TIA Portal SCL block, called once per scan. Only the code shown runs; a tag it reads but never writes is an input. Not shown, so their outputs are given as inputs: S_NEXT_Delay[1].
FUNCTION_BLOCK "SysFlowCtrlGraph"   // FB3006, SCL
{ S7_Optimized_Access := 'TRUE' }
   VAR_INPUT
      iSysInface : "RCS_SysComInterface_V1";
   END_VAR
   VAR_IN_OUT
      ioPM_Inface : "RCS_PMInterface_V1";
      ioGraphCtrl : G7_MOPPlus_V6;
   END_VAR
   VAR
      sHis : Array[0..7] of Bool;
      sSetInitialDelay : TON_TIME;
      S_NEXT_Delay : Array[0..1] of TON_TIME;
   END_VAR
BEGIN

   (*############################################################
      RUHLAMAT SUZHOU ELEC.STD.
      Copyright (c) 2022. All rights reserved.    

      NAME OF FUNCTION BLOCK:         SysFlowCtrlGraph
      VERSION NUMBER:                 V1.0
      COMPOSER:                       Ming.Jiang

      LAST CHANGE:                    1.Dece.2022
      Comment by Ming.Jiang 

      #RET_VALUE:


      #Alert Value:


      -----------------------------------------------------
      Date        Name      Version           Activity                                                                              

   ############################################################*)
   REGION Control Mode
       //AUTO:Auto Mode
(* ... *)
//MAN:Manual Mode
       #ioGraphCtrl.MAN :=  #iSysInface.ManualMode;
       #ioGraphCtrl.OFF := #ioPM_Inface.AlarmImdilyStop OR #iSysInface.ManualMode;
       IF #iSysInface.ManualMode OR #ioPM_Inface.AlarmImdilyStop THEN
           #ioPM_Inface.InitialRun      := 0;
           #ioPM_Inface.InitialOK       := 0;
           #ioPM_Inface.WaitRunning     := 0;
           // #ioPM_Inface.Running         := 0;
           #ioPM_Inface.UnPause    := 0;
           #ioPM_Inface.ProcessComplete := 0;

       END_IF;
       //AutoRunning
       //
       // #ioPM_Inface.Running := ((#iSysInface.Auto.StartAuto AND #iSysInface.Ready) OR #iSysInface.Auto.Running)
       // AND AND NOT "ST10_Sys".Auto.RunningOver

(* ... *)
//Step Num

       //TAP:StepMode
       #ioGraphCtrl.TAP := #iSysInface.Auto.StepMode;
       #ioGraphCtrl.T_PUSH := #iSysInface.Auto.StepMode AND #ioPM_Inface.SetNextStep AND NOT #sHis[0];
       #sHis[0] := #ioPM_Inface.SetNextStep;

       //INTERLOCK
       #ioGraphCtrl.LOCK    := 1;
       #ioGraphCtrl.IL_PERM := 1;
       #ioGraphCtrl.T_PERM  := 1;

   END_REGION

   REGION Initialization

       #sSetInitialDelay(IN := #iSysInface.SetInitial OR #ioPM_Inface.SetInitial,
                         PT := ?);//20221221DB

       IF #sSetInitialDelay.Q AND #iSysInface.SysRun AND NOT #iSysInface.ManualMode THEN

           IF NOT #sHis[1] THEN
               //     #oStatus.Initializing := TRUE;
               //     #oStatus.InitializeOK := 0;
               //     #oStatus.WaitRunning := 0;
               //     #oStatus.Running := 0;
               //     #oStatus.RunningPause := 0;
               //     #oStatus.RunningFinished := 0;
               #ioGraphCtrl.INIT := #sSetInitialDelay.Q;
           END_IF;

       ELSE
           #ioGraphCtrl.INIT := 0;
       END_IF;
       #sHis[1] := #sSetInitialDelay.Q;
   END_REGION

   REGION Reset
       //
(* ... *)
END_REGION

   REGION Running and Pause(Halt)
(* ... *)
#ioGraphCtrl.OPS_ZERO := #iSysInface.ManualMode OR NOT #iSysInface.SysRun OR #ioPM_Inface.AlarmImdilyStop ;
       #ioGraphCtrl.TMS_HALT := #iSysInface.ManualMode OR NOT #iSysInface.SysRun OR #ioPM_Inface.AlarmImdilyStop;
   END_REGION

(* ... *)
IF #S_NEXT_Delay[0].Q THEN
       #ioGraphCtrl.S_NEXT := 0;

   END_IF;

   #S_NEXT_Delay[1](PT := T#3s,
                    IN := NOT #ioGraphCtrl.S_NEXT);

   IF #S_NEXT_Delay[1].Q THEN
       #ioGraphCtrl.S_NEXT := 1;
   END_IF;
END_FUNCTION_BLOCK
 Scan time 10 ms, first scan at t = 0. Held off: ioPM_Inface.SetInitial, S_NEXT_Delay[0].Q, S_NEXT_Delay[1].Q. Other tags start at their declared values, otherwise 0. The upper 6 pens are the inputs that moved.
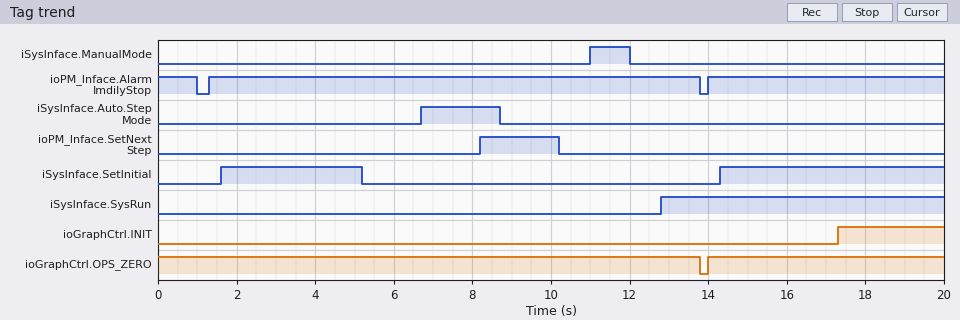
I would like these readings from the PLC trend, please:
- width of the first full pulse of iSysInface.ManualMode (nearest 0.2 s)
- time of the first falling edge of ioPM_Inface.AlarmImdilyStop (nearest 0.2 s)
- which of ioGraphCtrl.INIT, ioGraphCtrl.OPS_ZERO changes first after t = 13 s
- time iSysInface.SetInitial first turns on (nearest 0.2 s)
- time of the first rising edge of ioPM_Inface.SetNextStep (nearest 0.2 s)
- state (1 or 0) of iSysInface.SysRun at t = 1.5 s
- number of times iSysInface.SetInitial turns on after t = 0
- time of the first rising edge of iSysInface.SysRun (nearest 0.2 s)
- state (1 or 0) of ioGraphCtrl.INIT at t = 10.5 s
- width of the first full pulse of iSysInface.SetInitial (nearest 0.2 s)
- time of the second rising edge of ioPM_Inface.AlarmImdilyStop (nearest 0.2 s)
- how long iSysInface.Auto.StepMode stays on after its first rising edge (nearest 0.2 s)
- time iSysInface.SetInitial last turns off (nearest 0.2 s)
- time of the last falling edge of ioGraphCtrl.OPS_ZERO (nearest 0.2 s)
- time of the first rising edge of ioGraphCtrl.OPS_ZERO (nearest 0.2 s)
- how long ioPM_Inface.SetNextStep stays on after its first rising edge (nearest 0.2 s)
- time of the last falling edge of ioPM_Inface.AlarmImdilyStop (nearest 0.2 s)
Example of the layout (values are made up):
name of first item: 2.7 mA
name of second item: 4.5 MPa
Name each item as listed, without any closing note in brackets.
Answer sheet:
width of the first full pulse of iSysInface.ManualMode: 1.0 s
time of the first falling edge of ioPM_Inface.AlarmImdilyStop: 1.0 s
which of ioGraphCtrl.INIT, ioGraphCtrl.OPS_ZERO changes first after t = 13 s: ioGraphCtrl.OPS_ZERO
time iSysInface.SetInitial first turns on: 1.6 s
time of the first rising edge of ioPM_Inface.SetNextStep: 8.2 s
state (1 or 0) of iSysInface.SysRun at t = 1.5 s: 0
number of times iSysInface.SetInitial turns on after t = 0: 2
time of the first rising edge of iSysInface.SysRun: 12.8 s
state (1 or 0) of ioGraphCtrl.INIT at t = 10.5 s: 0
width of the first full pulse of iSysInface.SetInitial: 3.6 s
time of the second rising edge of ioPM_Inface.AlarmImdilyStop: 14.0 s
how long iSysInface.Auto.StepMode stays on after its first rising edge: 2.0 s
time iSysInface.SetInitial last turns off: 5.2 s
time of the last falling edge of ioGraphCtrl.OPS_ZERO: 13.8 s
time of the first rising edge of ioGraphCtrl.OPS_ZERO: 14.0 s
how long ioPM_Inface.SetNextStep stays on after its first rising edge: 2.0 s
time of the last falling edge of ioPM_Inface.AlarmImdilyStop: 13.8 s
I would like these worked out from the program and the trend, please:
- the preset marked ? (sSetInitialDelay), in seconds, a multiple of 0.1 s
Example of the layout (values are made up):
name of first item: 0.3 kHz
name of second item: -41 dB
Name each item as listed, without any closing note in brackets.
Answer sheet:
the preset marked ? (sSetInitialDelay), in seconds, a multiple of 0.1 s: 3.0 s
